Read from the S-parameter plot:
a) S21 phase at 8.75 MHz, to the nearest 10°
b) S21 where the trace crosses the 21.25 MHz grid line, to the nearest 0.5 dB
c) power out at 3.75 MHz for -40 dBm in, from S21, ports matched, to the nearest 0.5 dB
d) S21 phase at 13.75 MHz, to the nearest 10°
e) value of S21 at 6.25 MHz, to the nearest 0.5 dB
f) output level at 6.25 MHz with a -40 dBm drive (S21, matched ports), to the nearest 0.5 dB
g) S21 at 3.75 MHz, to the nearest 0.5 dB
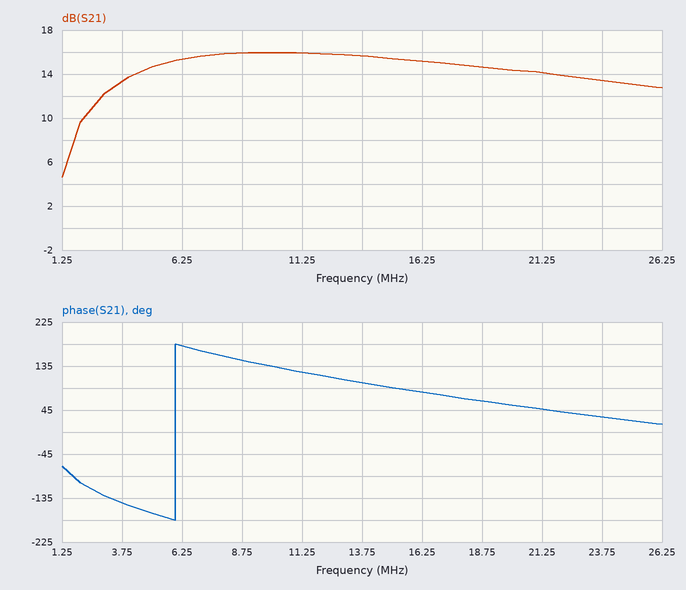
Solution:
150°
14.0 dB
-26.5 dBm
100°
15.5 dB
-24.5 dBm
13.5 dB
